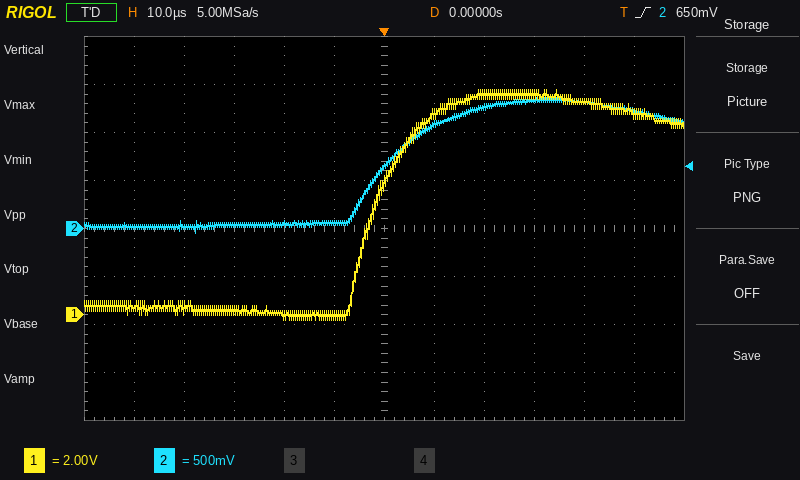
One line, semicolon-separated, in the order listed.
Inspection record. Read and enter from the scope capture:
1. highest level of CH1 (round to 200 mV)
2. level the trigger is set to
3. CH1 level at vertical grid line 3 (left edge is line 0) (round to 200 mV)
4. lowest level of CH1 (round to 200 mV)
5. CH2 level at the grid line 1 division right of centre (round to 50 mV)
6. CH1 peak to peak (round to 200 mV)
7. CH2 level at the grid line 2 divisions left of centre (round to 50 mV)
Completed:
9.4 V; 650 mV; 200 mV; -200 mV; 1.10 V; 9.6 V; 50 mV
